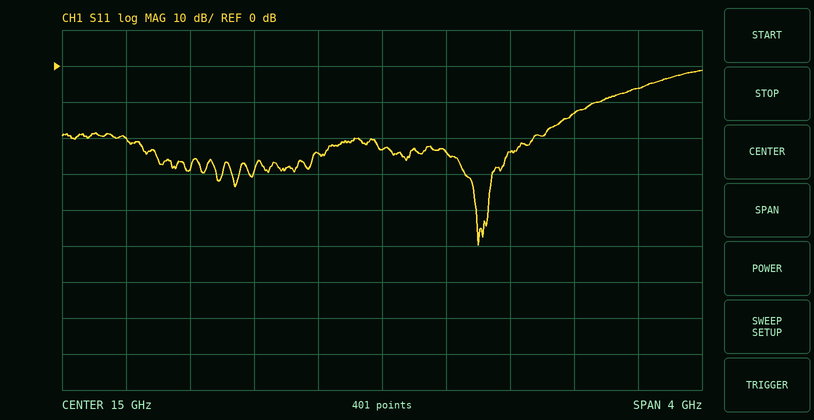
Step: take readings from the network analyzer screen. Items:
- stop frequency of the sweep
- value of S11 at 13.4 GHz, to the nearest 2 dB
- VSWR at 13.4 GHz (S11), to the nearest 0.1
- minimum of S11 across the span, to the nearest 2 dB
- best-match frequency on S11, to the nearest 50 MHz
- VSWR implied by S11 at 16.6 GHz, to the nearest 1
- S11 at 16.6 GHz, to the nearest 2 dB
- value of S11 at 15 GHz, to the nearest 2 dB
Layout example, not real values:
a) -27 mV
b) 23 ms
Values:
a) 17 GHz
b) -20 dB
c) 1.2
d) -50 dB
e) 15.60 GHz
f) 3
g) -6 dB
h) -24 dB
